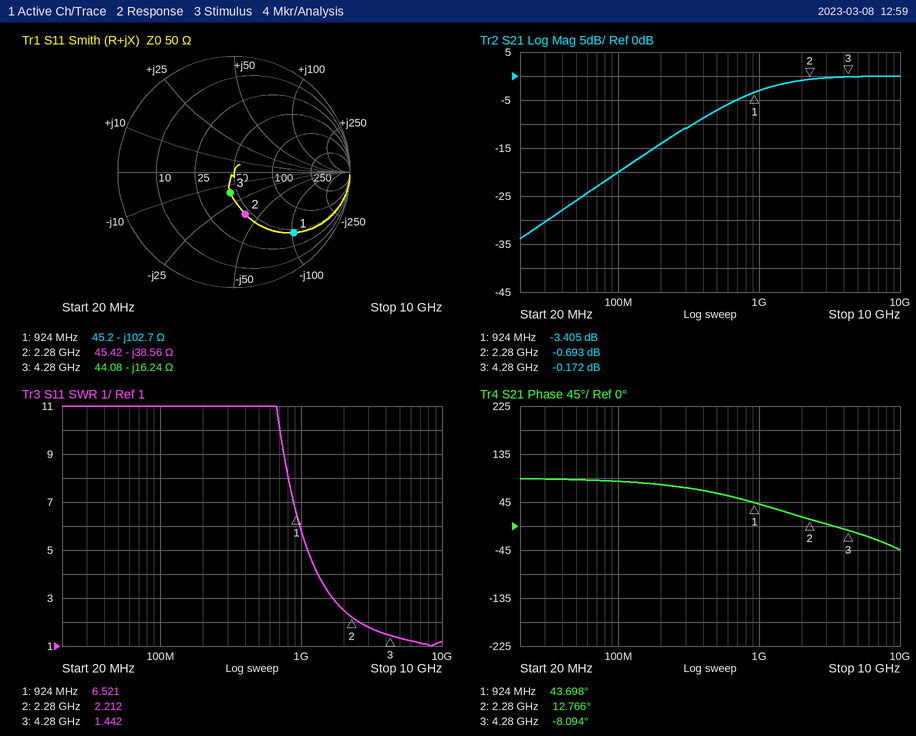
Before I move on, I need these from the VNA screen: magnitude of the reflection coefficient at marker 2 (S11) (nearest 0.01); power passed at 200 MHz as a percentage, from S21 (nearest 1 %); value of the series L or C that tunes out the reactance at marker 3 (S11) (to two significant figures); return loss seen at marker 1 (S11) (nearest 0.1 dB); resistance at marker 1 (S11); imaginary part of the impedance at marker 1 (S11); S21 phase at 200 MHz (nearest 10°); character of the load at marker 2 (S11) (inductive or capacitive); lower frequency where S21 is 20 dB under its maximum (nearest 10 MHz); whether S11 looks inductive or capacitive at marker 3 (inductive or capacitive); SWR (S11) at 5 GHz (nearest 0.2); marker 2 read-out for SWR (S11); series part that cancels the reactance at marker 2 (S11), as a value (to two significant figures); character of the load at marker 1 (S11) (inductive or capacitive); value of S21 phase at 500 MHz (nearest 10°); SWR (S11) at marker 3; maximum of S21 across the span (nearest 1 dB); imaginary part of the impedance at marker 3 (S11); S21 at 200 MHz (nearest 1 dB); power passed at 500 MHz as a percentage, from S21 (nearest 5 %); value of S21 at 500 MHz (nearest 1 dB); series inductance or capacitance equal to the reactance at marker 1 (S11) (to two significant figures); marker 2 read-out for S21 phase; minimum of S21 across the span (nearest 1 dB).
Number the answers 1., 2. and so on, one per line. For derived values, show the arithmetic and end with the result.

1. 0.38
2. 10^(-14/10) ≈ 4 %
3. L = 16.24 Ω/(2π × 4.28 GHz) ≈ 604 pH, so 600 pH to two significant figures
4. 2.7 dB
5. 45.2 Ω
6. -102.7 Ω
7. 80°
8. capacitive
9. 100 MHz
10. capacitive
11. 1.4
12. 2.212
13. L = 38.56 Ω/(2π × 2.28 GHz) ≈ 2.7 nH
14. capacitive
15. 60°
16. 1.442
17. 0 dB
18. -16.24 Ω
19. -14 dB
20. 10^(-7/10) ≈ 20 %
21. -7 dB
22. C = 1/(2π × 924 MHz × 102.7 Ω) ≈ 1.7 pF
23. 12.766°
24. -34 dB
